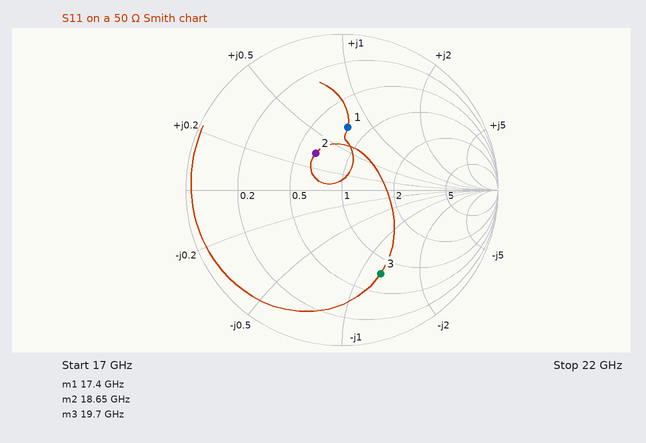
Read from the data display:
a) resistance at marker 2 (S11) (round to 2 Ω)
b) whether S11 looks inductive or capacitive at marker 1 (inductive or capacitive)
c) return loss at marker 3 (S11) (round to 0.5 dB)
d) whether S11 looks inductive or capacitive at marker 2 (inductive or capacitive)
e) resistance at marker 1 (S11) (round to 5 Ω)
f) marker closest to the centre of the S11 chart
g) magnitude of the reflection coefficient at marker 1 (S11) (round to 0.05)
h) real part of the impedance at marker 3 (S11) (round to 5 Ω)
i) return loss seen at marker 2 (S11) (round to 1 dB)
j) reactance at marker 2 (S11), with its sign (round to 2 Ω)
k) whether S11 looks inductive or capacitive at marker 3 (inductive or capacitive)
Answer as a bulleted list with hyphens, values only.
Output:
- 32 Ω
- inductive
- 4.5 dB
- inductive
- 40 Ω
- marker 2
- 0.40
- 40 Ω
- 11 dB
- +16 Ω
- capacitive
